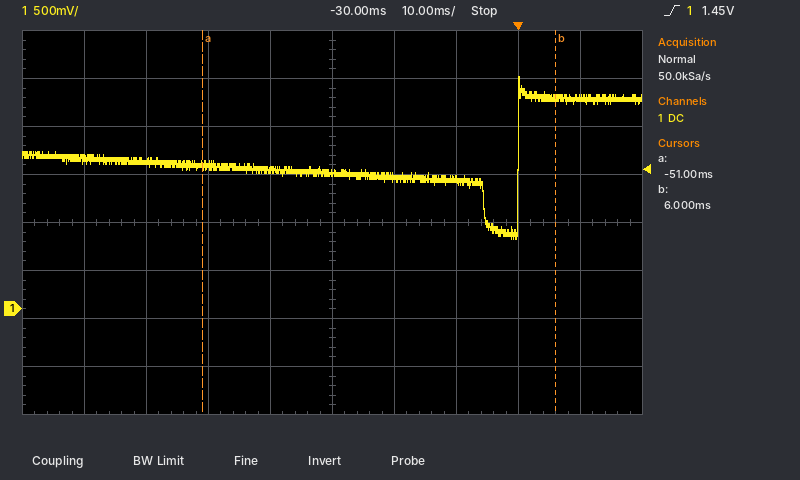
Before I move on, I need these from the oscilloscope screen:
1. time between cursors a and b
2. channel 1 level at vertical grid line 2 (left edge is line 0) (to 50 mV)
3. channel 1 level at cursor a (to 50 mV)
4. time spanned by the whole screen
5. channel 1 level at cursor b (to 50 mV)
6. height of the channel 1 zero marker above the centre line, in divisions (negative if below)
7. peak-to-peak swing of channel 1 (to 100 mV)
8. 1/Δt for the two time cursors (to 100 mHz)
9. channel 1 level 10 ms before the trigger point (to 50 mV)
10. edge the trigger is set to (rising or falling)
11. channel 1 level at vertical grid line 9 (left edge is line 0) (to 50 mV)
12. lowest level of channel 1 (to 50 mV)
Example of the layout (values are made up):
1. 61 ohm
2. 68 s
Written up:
1. 57 ms
2. 1.55 V
3. 1.50 V
4. 100 ms
5. 2.20 V
6. -1.8 div
7. 1.70 V
8. 17.5 Hz
9. 1.35 V
10. rising
11. 2.20 V
12. 750 mV
